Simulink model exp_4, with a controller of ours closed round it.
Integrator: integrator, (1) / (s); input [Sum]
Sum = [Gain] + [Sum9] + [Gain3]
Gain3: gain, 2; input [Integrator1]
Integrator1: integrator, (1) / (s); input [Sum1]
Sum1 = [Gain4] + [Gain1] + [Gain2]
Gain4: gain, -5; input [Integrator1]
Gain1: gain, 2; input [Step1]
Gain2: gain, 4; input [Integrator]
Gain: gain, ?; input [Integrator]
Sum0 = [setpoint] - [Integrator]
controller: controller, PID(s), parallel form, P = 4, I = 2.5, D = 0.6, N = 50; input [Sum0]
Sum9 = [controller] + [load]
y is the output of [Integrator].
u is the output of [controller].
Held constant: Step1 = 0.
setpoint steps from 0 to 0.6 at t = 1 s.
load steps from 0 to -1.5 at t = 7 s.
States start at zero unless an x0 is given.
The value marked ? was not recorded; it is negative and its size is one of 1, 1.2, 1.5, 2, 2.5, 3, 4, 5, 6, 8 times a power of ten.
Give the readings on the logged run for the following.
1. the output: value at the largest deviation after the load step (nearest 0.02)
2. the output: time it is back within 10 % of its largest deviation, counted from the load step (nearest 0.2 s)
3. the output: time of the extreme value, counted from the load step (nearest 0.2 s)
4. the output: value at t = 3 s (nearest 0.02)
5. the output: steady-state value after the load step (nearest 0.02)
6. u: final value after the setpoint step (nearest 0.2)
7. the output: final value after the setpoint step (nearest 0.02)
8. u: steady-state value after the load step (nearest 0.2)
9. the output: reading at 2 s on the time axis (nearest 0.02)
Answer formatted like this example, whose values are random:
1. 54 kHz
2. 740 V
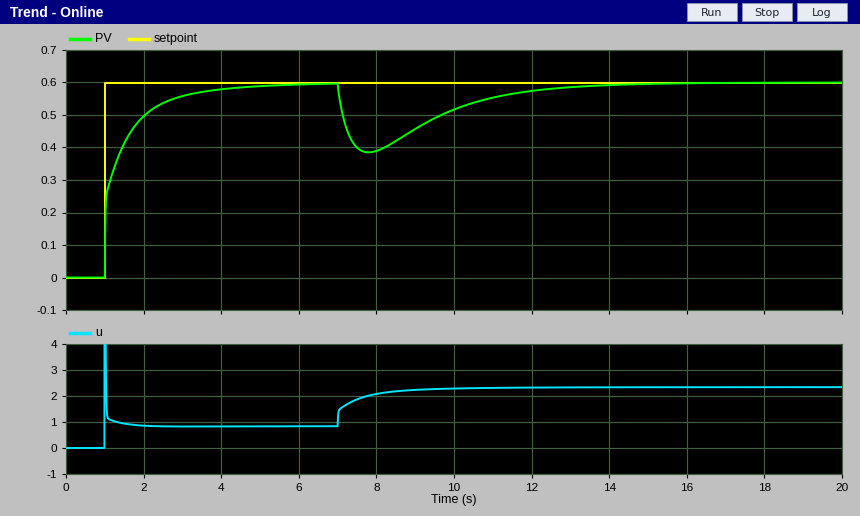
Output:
1. 0.38
2. 5.4 s
3. 0.8 s
4. 0.56
5. 0.60
6. 0.8
7. 0.60
8. 2.4
9. 0.50
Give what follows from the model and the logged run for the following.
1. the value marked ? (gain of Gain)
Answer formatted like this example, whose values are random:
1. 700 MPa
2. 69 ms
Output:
1. -3
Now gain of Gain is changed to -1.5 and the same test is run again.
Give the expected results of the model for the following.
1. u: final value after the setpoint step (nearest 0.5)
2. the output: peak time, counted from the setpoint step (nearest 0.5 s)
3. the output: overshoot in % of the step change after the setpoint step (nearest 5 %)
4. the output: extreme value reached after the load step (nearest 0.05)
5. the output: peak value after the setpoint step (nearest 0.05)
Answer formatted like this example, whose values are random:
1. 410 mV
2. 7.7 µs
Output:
1. 0.0
2. 2.0 s
3. 10 %
4. 0.35
5. 0.65
